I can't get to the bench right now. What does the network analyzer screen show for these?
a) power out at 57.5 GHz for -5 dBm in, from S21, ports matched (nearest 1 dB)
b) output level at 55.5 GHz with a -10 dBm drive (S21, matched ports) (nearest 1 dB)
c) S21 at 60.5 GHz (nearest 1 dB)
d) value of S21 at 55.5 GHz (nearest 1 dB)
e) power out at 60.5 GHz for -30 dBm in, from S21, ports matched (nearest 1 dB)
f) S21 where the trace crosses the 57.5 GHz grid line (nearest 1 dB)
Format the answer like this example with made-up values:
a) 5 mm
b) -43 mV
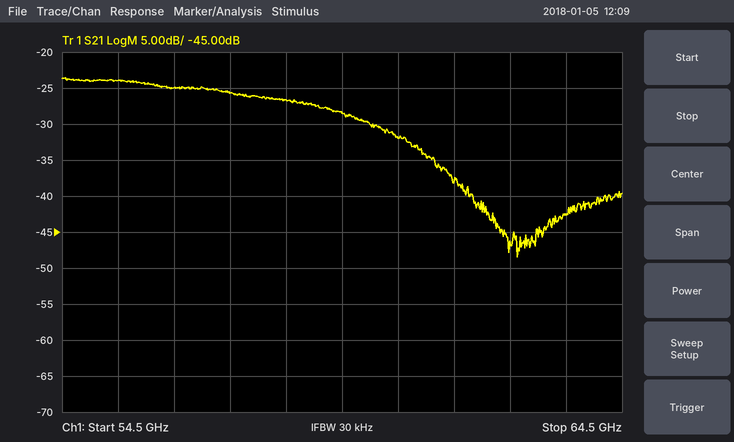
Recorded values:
a) -31 dBm
b) -34 dBm
c) -32 dB
d) -24 dB
e) -62 dBm
f) -26 dB
